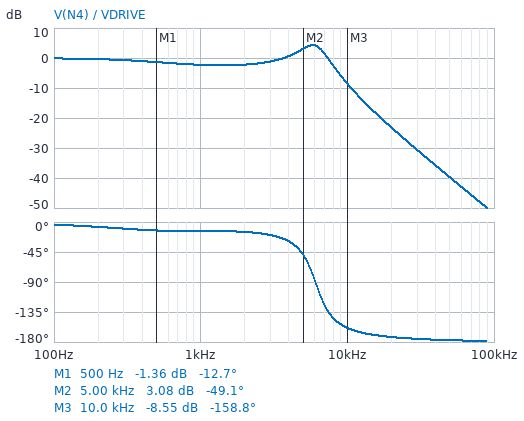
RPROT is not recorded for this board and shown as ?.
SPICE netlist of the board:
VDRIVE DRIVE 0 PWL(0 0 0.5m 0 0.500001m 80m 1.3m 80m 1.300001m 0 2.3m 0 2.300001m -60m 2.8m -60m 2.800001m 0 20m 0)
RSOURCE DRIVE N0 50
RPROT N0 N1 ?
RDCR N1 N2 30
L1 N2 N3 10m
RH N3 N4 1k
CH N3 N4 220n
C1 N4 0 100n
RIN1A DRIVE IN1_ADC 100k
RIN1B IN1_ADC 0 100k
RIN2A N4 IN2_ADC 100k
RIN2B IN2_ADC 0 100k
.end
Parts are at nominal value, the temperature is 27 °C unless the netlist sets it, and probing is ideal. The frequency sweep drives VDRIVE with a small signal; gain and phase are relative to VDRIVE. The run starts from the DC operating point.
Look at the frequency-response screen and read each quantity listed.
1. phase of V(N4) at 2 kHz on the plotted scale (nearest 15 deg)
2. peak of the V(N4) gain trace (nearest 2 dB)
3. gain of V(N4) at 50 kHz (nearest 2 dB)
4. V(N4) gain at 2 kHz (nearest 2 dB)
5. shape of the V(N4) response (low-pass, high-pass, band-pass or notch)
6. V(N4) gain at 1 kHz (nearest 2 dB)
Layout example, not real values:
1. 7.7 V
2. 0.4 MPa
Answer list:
1. -15 deg
2. 4 dB
3. -40 dB
4. -2 dB
5. low-pass
6. -2 dB
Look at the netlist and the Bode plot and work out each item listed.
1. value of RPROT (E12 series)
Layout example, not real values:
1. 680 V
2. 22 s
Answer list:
1. 68 Ω
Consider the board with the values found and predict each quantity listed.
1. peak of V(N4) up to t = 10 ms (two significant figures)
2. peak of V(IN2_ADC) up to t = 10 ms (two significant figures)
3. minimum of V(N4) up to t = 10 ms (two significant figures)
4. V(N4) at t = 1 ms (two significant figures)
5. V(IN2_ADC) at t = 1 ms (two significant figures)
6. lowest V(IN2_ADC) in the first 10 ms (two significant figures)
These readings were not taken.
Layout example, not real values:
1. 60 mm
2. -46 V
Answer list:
1. 87 mV
2. 43 mV
3. -64 mV
4. 73 mV
5. 37 mV
6. -32 mV
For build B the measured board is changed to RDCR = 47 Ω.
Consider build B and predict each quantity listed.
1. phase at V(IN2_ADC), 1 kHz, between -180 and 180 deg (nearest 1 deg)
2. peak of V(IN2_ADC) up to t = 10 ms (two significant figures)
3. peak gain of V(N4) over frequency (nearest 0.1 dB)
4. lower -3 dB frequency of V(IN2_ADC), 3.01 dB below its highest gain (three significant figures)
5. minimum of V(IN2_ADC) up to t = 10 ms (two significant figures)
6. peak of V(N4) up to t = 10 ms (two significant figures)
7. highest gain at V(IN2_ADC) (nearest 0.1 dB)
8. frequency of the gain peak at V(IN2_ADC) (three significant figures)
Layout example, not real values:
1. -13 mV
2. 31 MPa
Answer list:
1. -14 deg
2. 42 mV
3. 3.5 dB
4. 4.01 kHz
5. -31 mV
6. 85 mV
7. -2.5 dB
8. 5.76 kHz
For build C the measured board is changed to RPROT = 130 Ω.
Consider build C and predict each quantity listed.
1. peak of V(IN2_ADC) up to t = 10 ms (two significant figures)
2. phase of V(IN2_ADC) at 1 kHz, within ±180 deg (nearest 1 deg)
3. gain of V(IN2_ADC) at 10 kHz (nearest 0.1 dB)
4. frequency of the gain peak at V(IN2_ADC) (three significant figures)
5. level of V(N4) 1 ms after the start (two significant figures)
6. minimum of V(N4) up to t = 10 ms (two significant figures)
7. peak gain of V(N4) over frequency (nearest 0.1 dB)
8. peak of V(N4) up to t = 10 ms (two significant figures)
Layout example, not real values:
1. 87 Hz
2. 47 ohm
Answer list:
1. 40 mV
2. -15 deg
3. -15.1 dB
4. 5.57 kHz
5. 74 mV
6. -59 mV
7. 1.7 dB
8. 80 mV
